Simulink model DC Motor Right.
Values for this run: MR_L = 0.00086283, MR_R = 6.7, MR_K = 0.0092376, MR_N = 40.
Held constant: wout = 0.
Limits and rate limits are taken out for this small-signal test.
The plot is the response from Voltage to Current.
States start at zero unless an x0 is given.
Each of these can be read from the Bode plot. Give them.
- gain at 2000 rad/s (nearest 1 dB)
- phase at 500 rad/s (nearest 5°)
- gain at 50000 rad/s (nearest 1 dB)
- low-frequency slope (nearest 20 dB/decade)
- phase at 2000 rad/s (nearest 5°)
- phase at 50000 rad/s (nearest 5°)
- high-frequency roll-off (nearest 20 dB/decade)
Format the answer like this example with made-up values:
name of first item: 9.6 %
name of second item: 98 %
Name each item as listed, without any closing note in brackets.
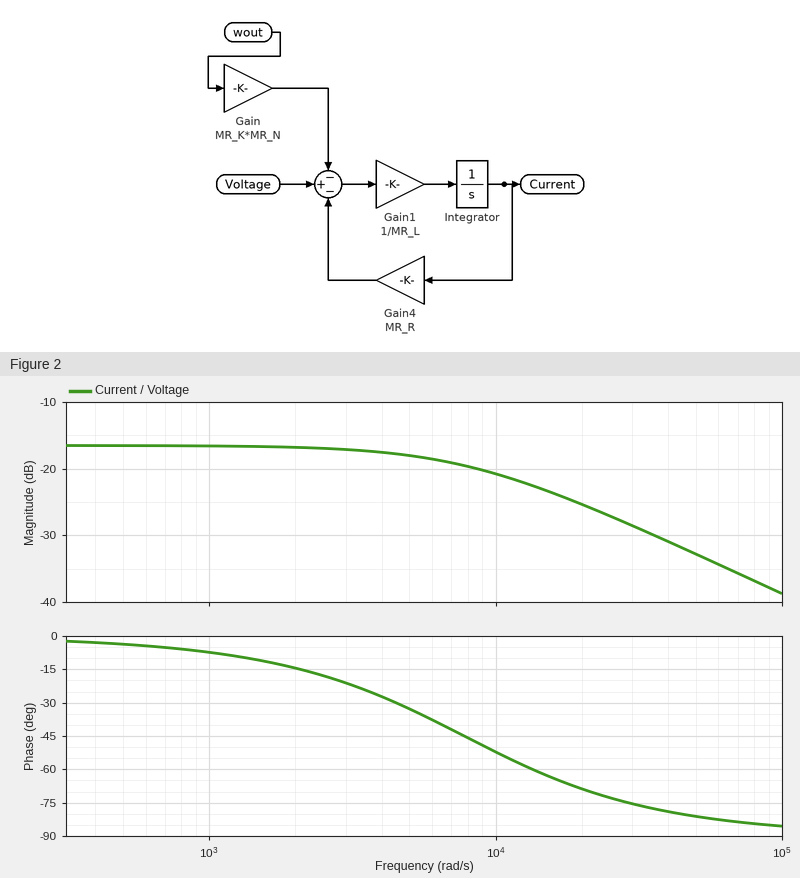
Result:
gain at 2000 rad/s: -17 dB
phase at 500 rad/s: -5°
gain at 50000 rad/s: -33 dB
low-frequency slope: 0 dB/decade
phase at 2000 rad/s: -15°
phase at 50000 rad/s: -80°
high-frequency roll-off: -20 dB/decade
